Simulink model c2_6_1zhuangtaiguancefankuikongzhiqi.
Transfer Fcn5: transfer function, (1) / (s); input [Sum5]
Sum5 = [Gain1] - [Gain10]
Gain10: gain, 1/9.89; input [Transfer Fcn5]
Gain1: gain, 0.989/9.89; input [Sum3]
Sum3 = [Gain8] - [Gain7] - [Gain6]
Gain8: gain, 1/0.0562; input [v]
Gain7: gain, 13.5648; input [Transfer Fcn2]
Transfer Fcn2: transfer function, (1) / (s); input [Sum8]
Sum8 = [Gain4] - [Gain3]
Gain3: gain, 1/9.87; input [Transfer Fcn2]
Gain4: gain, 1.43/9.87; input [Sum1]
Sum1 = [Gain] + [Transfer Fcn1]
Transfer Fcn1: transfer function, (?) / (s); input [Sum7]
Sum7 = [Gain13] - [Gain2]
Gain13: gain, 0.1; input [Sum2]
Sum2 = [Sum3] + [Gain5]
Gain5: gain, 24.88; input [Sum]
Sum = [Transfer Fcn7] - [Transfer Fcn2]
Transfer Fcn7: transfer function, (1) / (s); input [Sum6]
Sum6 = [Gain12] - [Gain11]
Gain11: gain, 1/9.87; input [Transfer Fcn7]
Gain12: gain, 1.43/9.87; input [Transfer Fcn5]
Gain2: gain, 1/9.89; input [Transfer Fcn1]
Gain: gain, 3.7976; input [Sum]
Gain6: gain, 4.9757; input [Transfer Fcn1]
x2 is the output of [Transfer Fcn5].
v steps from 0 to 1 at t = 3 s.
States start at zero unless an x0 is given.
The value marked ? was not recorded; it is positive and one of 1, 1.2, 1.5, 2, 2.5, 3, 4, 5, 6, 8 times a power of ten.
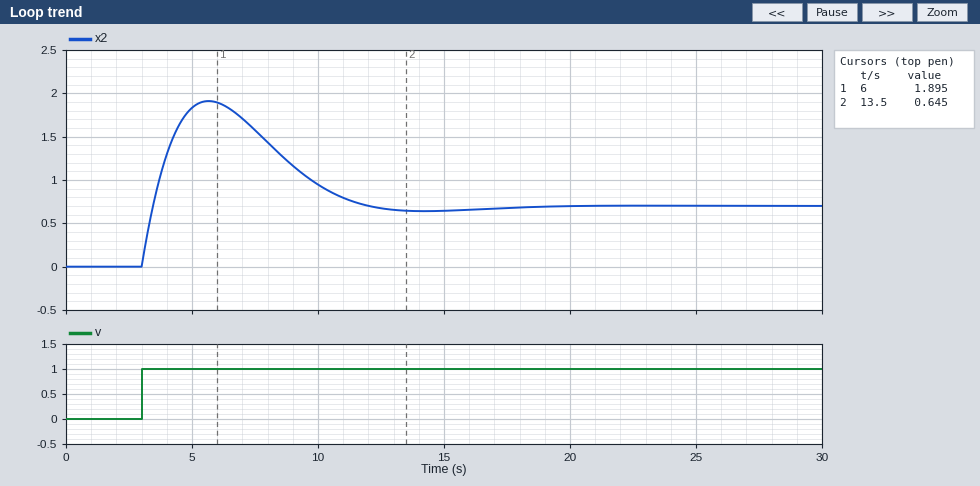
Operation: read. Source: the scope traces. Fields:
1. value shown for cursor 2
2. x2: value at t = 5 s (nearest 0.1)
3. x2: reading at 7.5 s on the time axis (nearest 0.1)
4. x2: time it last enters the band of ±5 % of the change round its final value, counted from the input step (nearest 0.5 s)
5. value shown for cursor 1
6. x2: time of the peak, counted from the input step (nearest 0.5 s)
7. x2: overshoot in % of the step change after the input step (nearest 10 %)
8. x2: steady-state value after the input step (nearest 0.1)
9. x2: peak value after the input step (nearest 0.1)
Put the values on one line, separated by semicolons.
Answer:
0.645; 1.8; 1.6; 13.5 s; 1.895; 2.5 s; 170 %; 0.7; 1.9
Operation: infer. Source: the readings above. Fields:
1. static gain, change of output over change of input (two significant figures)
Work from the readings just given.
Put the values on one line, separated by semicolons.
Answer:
0.70
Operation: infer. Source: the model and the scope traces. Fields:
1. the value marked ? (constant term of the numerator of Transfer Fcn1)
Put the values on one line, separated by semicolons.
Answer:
1
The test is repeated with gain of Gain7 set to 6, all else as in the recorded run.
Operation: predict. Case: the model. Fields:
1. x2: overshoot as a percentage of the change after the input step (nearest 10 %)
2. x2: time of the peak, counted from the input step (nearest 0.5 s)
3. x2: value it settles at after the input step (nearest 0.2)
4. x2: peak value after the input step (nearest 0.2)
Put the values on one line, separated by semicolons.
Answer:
80 %; 3.5 s; 1.2; 2.2
